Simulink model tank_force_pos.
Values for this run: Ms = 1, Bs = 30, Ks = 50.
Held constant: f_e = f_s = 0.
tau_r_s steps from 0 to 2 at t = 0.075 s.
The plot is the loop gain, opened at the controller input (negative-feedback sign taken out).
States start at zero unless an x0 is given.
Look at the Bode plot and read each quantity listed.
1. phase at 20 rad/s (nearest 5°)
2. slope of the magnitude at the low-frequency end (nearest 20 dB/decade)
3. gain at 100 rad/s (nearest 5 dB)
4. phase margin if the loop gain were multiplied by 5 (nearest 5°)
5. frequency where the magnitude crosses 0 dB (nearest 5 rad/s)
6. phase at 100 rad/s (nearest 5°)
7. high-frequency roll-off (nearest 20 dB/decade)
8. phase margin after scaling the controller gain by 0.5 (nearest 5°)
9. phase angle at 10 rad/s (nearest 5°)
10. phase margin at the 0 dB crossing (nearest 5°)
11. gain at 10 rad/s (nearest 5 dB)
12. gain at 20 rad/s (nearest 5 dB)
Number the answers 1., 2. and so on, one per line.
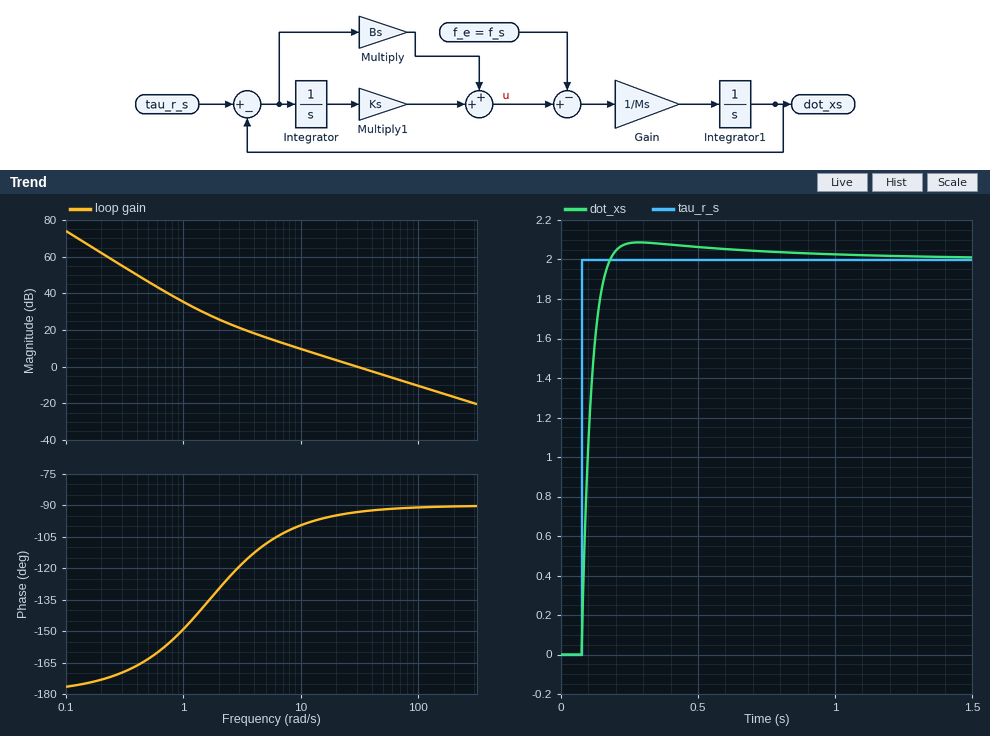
1. -95°
2. -40 dB/decade
3. -10 dB
4. 90°
5. 30 rad/s
6. -90°
7. -20 dB/decade
8. 85°
9. -100°
10. 85°
11. 10 dB
12. 5 dB
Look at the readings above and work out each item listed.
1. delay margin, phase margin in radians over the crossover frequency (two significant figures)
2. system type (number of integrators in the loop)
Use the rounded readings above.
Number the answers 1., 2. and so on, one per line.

1. 0.049 s
2. 2
